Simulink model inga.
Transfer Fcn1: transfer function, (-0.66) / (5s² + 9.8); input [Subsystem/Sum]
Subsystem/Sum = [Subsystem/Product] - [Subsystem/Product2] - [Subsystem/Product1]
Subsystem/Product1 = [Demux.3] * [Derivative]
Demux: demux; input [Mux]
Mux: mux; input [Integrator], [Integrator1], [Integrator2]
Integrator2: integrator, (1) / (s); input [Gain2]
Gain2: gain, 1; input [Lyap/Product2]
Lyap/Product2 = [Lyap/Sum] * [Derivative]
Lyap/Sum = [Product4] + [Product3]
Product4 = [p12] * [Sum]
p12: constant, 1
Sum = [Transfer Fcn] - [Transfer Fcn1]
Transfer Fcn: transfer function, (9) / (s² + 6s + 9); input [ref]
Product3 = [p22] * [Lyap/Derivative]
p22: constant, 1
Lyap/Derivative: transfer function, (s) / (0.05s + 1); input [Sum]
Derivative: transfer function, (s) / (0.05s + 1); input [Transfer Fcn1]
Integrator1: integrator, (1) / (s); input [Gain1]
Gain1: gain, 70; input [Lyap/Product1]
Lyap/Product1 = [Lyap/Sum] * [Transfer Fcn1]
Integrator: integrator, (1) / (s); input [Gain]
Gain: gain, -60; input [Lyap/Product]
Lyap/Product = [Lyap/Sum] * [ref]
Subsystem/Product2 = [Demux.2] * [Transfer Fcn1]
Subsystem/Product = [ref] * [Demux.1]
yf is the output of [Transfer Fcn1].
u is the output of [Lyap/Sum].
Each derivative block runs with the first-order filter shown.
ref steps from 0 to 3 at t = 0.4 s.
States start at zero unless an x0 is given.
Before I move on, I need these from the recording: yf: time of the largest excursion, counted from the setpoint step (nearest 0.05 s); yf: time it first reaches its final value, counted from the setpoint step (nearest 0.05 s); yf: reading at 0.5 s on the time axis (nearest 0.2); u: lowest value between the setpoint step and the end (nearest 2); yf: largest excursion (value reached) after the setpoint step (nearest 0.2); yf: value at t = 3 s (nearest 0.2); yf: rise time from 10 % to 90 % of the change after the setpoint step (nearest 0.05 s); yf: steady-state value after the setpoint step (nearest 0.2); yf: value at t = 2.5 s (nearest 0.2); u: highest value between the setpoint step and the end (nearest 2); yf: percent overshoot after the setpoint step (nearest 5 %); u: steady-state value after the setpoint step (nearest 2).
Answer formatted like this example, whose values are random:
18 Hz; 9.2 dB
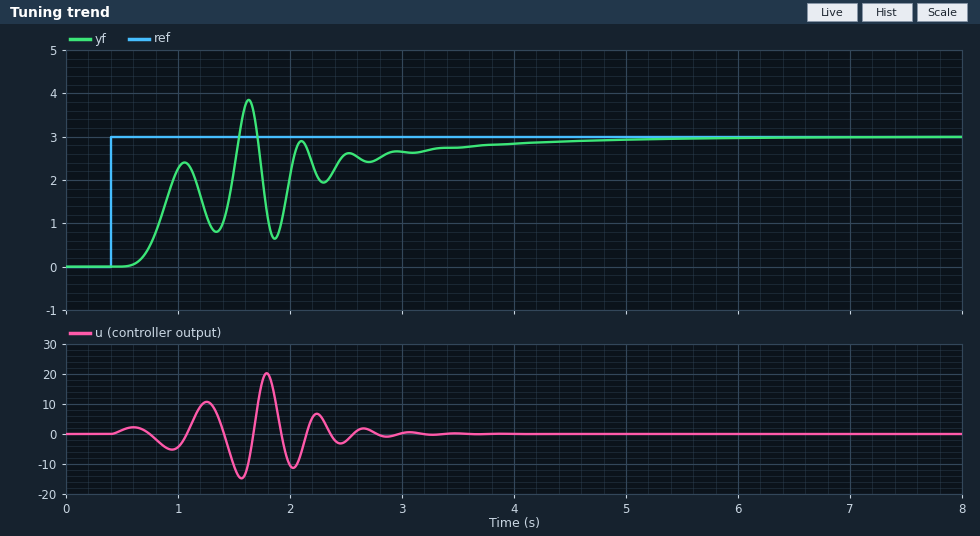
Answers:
1.25 s; 1.15 s; 0.0; -14; 3.8; 2.6; 0.80 s; 3.0; 2.6; 20; 30 %; 0
